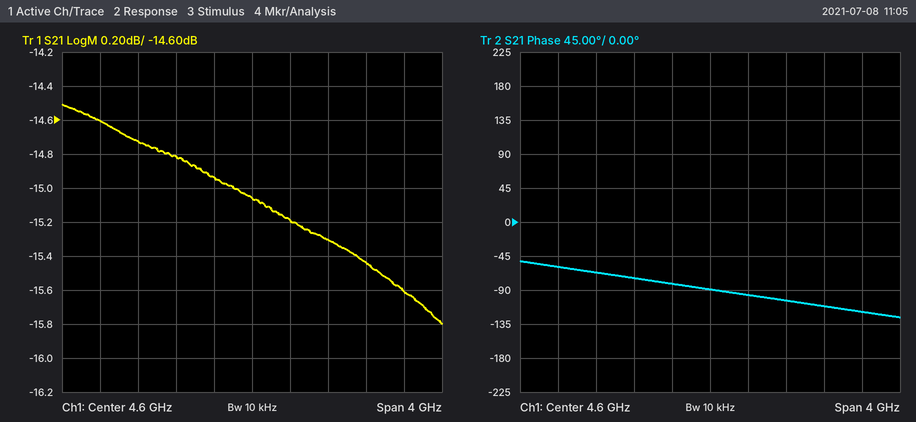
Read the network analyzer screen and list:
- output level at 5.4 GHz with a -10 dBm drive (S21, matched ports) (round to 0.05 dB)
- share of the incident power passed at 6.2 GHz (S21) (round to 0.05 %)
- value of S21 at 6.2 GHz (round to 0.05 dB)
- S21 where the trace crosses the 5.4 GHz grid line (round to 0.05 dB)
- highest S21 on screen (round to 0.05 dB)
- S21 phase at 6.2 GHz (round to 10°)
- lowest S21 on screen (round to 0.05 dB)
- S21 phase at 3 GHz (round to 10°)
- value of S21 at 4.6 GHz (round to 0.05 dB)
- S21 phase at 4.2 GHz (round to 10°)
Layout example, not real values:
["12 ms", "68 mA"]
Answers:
["-25.30 dBm", "2.75 %", "-15.60 dB", "-15.30 dB", "-14.50 dB", "-120°", "-15.80 dB", "-60°", "-15.05 dB", "-80°"]
